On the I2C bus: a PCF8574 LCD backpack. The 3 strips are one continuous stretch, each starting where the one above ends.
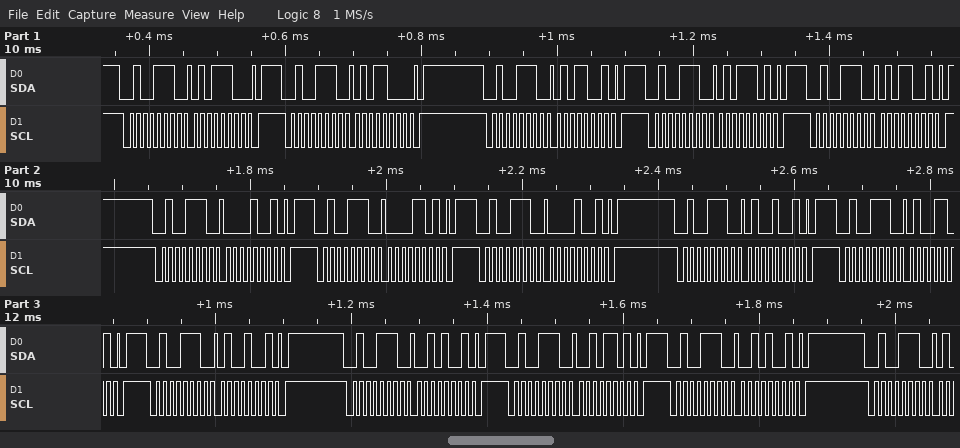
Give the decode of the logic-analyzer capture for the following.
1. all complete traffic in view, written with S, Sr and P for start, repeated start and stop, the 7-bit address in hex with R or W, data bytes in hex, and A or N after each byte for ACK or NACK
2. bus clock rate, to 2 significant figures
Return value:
S 27W A 5C A P S 27W A 58 A P S 27W A 59 A P S 27W A 5D A P S 27W A 59 A P S 27W A 09 A P S 27W A 0D A P S 27W A 09 A P S 27W A 49 A P S 27W A 4D A P S 27W A 49 A P S 27W A 29 A P S 27W A 2D A P S 27W A 29 A P S 27W A
100 kHz
